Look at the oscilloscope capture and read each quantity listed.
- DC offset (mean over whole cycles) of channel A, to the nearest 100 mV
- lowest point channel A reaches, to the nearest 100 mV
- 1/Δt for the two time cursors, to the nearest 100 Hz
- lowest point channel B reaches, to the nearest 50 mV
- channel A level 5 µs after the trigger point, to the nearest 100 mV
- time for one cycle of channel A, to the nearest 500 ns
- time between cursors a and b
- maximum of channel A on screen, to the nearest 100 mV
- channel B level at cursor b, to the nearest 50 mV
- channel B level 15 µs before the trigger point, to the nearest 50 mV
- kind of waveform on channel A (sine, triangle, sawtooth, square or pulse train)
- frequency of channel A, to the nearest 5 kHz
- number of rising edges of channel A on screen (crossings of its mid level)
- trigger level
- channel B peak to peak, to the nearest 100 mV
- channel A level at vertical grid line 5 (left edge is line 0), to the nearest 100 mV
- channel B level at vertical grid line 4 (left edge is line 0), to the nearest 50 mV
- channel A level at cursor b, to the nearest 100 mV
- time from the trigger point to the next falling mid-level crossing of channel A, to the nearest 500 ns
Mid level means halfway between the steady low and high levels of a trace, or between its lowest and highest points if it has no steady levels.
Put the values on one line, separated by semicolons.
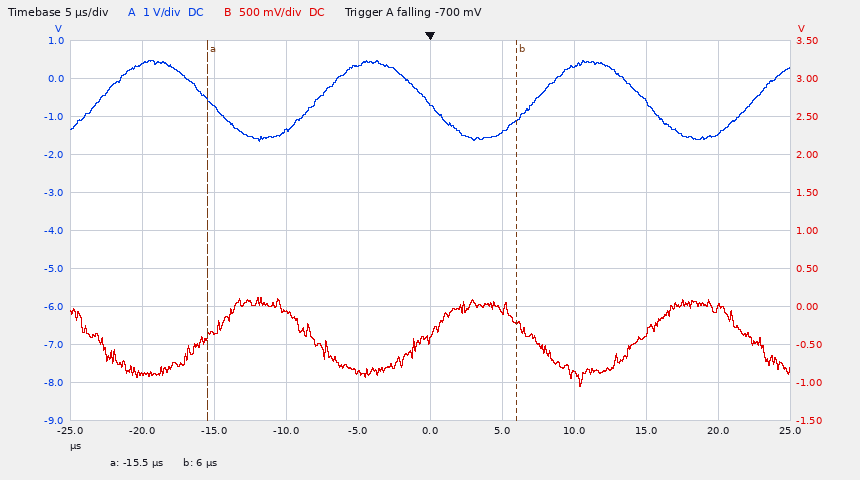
-600 mV; -1.7 V; 46.5 kHz; -1.05 V; -1.4 V; 15.0 µs; 21.5 µs; 500 mV; -200 mV; -350 mV; sine; 65 kHz; 4; -700 mV; 1.20 V; -700 mV; -850 mV; -1.1 V; 15.0 µs
